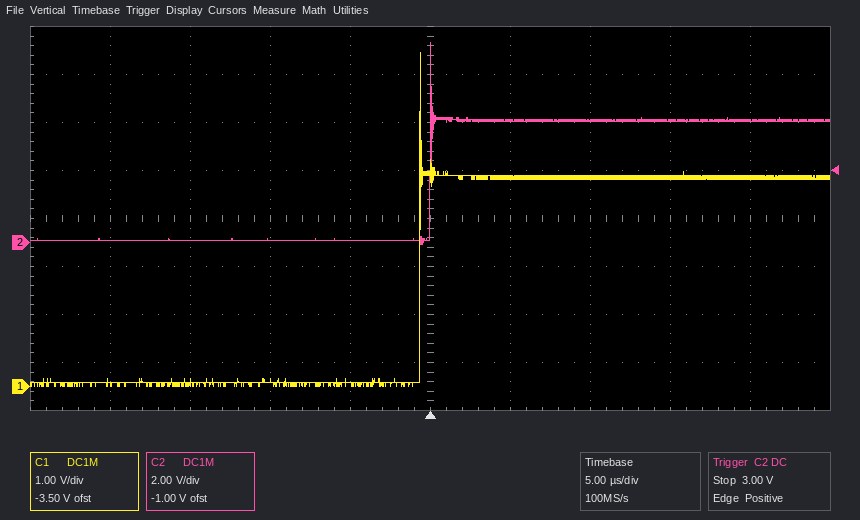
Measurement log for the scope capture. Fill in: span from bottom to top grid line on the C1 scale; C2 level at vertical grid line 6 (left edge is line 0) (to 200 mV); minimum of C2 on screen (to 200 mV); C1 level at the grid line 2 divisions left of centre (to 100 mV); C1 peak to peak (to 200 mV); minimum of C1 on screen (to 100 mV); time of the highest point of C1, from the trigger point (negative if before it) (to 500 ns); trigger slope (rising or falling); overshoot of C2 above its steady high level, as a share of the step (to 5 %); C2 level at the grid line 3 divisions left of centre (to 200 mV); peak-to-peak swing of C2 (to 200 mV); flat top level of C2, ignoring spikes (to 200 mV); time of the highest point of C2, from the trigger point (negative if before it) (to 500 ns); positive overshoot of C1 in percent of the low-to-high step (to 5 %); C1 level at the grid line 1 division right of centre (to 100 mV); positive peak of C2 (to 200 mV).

8 V
5.0 V
0.0 V
100 mV
7.0 V
0.0 V
-500 ns
rising
65 %
0.0 V
8.4 V
5.0 V
0.0 µs
60 %
4.4 V
8.4 V
